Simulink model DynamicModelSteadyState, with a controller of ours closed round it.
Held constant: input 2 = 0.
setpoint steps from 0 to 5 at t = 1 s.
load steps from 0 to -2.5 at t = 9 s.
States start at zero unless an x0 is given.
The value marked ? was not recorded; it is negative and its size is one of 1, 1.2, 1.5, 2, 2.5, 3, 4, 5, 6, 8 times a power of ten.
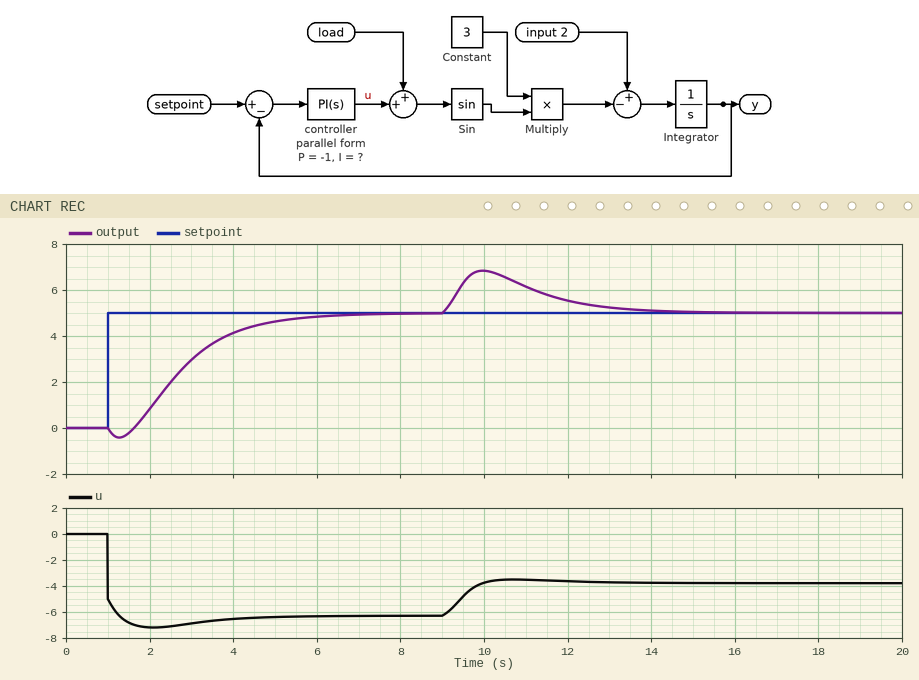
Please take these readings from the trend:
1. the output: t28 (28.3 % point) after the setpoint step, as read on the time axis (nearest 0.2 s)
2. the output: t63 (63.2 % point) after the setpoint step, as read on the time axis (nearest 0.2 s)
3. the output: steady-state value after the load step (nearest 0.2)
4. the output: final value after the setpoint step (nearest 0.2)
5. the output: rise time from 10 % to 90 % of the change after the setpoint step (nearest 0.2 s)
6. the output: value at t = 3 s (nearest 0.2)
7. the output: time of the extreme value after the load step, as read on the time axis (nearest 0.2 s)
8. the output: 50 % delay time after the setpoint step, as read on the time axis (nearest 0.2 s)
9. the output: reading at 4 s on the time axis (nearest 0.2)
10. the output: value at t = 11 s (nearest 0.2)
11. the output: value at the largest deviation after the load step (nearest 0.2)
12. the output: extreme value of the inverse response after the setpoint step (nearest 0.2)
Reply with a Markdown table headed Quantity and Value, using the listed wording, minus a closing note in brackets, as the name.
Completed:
| Quantity | Value |
|---|---|
| the output: t28 (28.3 % point) after the setpoint step, as read on the time axis | 2.2 s |
| the output: t63 (63.2 % point) after the setpoint step, as read on the time axis | 3.2 s |
| the output: steady-state value after the load step | 5.0 |
| the output: final value after the setpoint step | 5.0 |
| the output: rise time from 10 % to 90 % of the change after the setpoint step | 2.8 s |
| the output: value at t = 3 s | 3.0 |
| the output: time of the extreme value after the load step, as read on the time axis | 10.0 s |
| the output: 50 % delay time after the setpoint step, as read on the time axis | 2.8 s |
| the output: reading at 4 s on the time axis | 4.2 |
| the output: value at t = 11 s | 6.2 |
| the output: value at the largest deviation after the load step | 6.8 |
| the output: extreme value of the inverse response after the setpoint step | -0.4 |
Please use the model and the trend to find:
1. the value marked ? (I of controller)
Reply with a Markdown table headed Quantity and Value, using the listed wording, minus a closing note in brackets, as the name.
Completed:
| Quantity | Value |
|---|---|
| the value marked ? | -0.6 |
